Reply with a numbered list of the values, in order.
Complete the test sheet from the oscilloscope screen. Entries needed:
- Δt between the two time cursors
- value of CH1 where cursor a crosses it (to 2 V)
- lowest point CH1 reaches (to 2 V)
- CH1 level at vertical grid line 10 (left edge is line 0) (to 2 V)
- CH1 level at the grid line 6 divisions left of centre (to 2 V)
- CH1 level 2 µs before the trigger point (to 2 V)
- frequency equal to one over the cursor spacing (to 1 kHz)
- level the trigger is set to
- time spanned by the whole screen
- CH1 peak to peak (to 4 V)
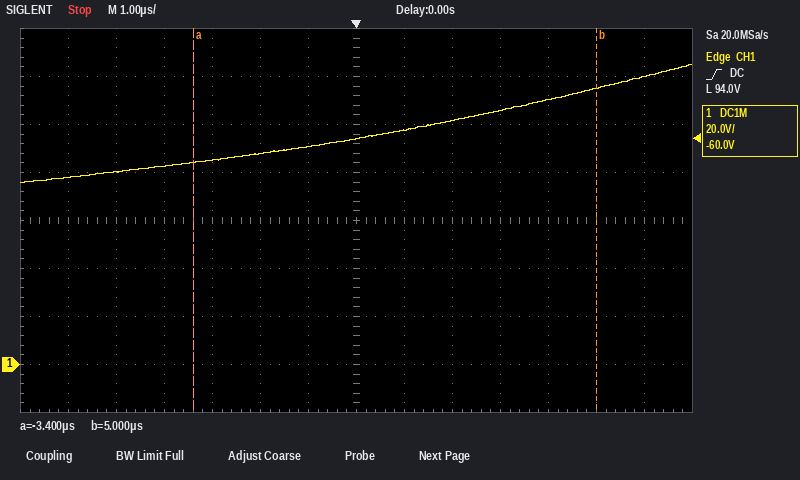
1. 8.4 µs
2. 84 V
3. 76 V
4. 106 V
5. 78 V
6. 88 V
7. 119 kHz
8. 94.0 V
9. 14 µs
10. 48 V
